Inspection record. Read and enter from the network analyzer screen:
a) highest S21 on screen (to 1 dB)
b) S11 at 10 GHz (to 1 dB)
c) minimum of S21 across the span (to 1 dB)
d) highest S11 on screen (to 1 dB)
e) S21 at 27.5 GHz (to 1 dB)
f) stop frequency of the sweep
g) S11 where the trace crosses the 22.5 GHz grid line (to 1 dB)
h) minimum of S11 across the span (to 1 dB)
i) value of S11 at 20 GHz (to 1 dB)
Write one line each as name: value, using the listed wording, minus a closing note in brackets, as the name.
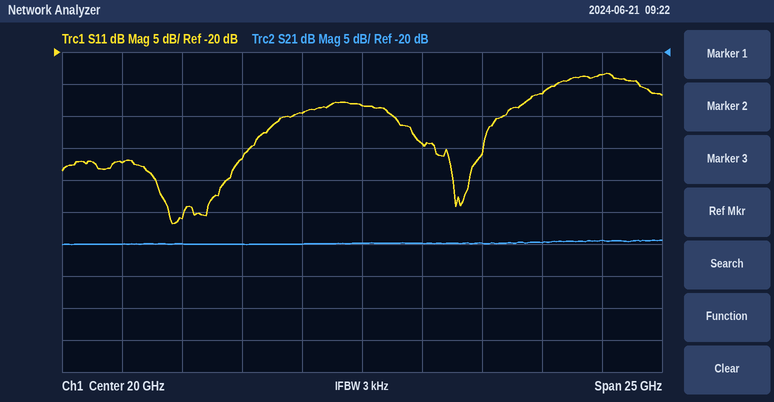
highest S21 on screen: -49 dB
S11 at 10 GHz: -37 dB
minimum of S21 across the span: -50 dB
highest S11 on screen: -23 dB
S21 at 27.5 GHz: -50 dB
stop frequency of the sweep: 32.5 GHz
S11 where the trace crosses the 22.5 GHz grid line: -34 dB
minimum of S11 across the span: -47 dB
value of S11 at 20 GHz: -28 dB
